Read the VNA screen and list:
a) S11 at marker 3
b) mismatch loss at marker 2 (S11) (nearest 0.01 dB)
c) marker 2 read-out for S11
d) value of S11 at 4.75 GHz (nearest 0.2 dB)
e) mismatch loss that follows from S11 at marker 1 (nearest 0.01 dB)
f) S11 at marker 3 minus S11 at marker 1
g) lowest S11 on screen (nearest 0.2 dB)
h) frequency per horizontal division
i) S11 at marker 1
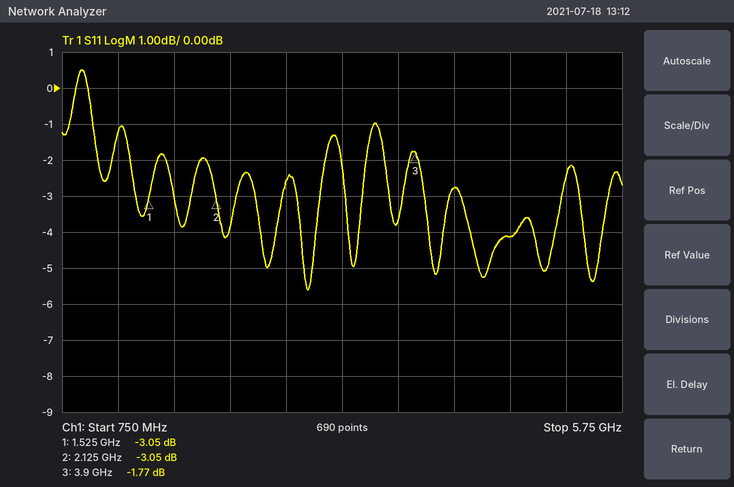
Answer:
-1.77 dB
2.97 dB
-3.05 dB
-4.2 dB
2.97 dB
1.28 dB
-5.6 dB
500 MHz
-3.05 dB
